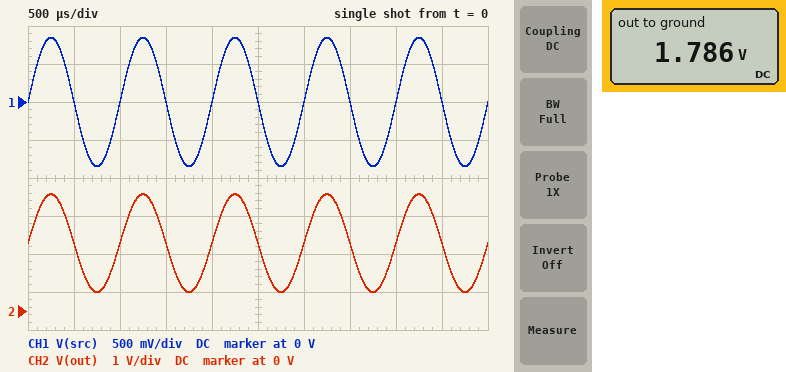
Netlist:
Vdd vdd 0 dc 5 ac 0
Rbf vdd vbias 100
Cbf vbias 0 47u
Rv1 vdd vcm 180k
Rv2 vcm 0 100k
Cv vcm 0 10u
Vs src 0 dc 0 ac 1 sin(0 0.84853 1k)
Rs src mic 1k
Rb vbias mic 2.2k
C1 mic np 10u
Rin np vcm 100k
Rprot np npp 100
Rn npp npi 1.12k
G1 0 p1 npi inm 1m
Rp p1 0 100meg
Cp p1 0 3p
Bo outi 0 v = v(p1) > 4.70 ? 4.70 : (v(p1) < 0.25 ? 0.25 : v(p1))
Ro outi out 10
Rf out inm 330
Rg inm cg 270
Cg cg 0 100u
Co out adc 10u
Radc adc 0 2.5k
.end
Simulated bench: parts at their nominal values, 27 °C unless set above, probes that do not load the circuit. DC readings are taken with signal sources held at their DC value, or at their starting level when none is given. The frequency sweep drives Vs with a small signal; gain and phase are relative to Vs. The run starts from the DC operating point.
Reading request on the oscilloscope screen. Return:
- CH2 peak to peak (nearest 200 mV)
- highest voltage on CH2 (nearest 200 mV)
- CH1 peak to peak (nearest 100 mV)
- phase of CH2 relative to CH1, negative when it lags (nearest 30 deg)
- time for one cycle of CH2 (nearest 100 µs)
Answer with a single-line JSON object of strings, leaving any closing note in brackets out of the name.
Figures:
{"CH2 peak to peak": "2.6 V", "highest voltage on CH2": "3.0 V", "CH1 peak to peak": "1.7 V", "phase of CH2 relative to CH1, negative when it lags": "0 deg", "time for one cycle of CH2": "1.0 ms"}
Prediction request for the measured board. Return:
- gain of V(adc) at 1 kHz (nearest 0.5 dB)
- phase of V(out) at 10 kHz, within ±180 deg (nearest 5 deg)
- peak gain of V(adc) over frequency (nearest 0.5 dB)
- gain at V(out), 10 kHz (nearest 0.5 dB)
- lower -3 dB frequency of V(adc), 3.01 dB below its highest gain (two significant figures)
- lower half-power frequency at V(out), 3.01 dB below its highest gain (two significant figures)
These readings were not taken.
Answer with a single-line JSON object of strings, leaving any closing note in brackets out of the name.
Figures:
{"gain of V(adc) at 1 kHz": "3.5 dB", "phase of V(out) at 10 kHz, within ±180 deg": "0 deg", "peak gain of V(adc) over frequency": "3.5 dB", "gain at V(out), 10 kHz": "3.5 dB", "lower -3 dB frequency of V(adc), 3.01 dB below its highest gain": "8.7 Hz", "lower half-power frequency at V(out), 3.01 dB below its highest gain": "4.4 Hz"}
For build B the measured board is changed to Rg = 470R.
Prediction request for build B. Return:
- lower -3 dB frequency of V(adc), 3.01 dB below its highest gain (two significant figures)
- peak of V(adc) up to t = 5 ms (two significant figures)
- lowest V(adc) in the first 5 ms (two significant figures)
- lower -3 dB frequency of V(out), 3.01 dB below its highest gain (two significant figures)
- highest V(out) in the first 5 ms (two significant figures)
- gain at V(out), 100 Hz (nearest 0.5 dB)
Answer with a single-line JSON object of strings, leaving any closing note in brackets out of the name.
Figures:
{"lower -3 dB frequency of V(adc), 3.01 dB below its highest gain": "7.1 Hz", "peak of V(adc) up to t = 5 ms": "980 mV", "lowest V(adc) in the first 5 ms": "-990 mV", "lower -3 dB frequency of V(out), 3.01 dB below its highest gain": "1.9 Hz", "highest V(out) in the first 5 ms": "2.8 V", "gain at V(out), 100 Hz": "1.5 dB"}
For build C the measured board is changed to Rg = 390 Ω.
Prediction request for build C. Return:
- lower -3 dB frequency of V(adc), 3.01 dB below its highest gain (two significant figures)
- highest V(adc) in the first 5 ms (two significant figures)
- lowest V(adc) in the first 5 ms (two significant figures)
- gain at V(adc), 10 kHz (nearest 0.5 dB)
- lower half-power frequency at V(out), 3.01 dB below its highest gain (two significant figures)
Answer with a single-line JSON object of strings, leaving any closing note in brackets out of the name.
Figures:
{"lower -3 dB frequency of V(adc), 3.01 dB below its highest gain": "7.5 Hz", "highest V(adc) in the first 5 ms": "1.1 V", "lowest V(adc) in the first 5 ms": "-1.1 V", "gain at V(adc), 10 kHz": "2.0 dB", "lower half-power frequency at V(out), 3.01 dB below its highest gain": "2.6 Hz"}
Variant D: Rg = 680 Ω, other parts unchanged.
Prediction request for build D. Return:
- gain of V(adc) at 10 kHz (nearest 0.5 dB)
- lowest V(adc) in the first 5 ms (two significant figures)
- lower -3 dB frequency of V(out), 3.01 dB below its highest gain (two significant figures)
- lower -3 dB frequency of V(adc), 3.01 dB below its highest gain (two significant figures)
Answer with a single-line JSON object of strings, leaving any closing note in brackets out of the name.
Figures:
{"gain of V(adc) at 10 kHz": "0 dB", "lowest V(adc) in the first 5 ms": "-870 mV", "lower -3 dB frequency of V(out), 3.01 dB below its highest gain": "940 mHz", "lower -3 dB frequency of V(adc), 3.01 dB below its highest gain": "6.6 Hz"}
